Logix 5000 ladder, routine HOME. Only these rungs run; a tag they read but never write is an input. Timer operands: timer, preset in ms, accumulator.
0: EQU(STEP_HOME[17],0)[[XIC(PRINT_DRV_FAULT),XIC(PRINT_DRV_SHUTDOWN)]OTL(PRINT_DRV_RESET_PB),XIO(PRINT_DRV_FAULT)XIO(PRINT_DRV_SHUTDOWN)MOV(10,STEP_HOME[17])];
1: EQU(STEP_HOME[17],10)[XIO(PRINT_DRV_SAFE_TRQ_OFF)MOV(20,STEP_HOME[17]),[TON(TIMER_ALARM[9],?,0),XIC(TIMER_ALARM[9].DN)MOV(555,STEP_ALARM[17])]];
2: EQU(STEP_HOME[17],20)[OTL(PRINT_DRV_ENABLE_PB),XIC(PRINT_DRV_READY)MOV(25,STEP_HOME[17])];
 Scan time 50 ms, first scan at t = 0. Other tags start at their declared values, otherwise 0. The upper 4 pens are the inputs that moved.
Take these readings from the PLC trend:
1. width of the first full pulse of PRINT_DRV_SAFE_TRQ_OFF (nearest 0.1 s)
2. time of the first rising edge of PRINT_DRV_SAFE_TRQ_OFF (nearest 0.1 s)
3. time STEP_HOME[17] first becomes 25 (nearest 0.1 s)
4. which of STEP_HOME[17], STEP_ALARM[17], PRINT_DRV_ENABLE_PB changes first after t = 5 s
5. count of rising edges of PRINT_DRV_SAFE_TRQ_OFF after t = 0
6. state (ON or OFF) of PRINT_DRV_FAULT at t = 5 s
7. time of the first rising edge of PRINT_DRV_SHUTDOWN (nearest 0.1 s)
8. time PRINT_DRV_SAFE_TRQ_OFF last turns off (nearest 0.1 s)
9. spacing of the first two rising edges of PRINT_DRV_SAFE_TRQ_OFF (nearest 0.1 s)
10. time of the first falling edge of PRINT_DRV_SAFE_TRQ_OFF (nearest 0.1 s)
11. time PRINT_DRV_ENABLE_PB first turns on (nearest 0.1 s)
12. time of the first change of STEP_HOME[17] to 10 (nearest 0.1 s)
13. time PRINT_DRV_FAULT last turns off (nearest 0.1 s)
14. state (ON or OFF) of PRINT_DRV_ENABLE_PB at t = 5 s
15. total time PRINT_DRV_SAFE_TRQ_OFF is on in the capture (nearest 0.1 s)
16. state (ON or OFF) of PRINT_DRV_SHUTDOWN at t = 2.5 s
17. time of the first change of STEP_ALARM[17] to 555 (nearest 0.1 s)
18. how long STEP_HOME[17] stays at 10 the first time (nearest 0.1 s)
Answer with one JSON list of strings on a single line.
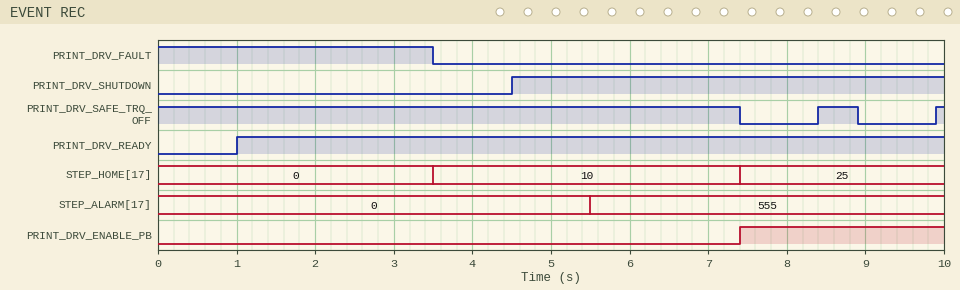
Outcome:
["0.5 s", "8.4 s", "7.4 s", "STEP_ALARM[17]", "2", "OFF", "4.5 s", "8.9 s", "1.5 s", "7.4 s", "7.4 s", "3.5 s", "3.5 s", "OFF", "8.0 s", "OFF", "5.5 s", "3.9 s"]
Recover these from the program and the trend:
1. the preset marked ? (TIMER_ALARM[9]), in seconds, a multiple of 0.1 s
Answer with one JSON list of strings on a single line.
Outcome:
["2.0 s"]
